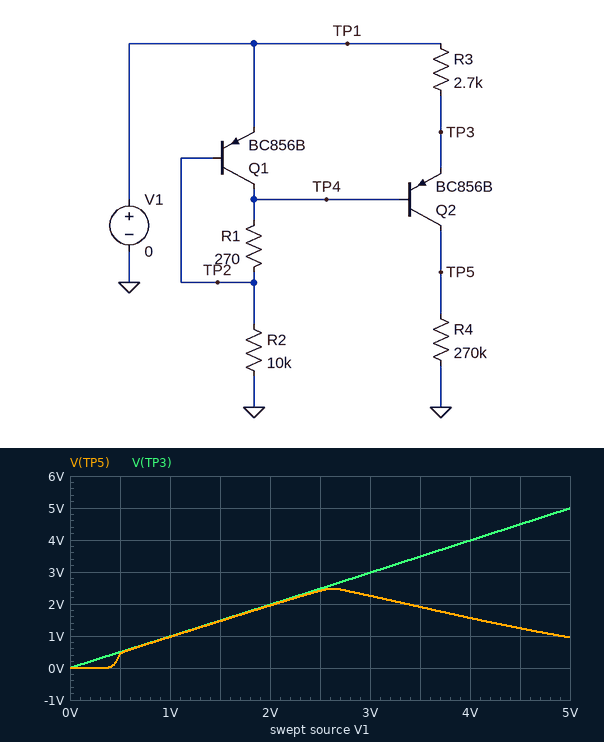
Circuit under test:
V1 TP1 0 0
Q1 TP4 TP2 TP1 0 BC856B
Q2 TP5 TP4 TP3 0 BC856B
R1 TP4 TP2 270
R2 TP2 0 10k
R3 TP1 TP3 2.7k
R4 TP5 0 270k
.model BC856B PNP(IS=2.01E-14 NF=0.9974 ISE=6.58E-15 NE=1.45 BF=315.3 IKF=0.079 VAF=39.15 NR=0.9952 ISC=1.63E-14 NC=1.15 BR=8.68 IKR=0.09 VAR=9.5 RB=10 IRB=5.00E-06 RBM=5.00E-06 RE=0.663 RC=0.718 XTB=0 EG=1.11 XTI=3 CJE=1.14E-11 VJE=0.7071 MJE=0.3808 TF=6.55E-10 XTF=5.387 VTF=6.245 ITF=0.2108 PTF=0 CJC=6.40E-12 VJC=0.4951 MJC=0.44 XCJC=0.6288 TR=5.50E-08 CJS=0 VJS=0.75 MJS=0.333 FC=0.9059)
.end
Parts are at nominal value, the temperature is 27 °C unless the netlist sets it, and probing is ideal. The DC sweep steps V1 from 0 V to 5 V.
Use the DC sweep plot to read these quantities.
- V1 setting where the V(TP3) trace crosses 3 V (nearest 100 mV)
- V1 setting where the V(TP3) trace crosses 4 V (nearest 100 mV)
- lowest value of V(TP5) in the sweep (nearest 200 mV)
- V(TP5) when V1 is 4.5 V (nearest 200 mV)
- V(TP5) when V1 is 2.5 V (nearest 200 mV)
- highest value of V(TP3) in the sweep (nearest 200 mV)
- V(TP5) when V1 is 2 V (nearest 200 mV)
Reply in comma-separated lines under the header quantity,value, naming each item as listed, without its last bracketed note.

quantity,value
V1 setting where the V(TP3) trace crosses 3 V,3.0 V
V1 setting where the V(TP3) trace crosses 4 V,4.0 V
lowest value of V(TP5) in the sweep,0 V
V(TP5) when V1 is 4.5 V,1.2 V
V(TP5) when V1 is 2.5 V,2.4 V
highest value of V(TP3) in the sweep,5.0 V
V(TP5) when V1 is 2 V,2.0 V
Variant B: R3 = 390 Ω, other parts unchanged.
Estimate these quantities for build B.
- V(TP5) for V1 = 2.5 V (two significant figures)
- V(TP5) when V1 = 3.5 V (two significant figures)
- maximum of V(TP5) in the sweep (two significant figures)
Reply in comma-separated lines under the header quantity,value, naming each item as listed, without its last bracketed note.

quantity,value
V(TP5) for V1 = 2.5 V,2.5 V
V(TP5) when V1 = 3.5 V,3.2 V
maximum of V(TP5) in the sweep,3.3 V
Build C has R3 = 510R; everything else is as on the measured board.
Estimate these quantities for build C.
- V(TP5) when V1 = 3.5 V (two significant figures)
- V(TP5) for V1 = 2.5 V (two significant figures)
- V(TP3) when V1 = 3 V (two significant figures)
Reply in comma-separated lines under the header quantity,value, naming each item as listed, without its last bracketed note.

quantity,value
V(TP5) when V1 = 3.5 V,3.1 V
V(TP5) for V1 = 2.5 V,2.5 V
V(TP3) when V1 = 3 V,3.0 V
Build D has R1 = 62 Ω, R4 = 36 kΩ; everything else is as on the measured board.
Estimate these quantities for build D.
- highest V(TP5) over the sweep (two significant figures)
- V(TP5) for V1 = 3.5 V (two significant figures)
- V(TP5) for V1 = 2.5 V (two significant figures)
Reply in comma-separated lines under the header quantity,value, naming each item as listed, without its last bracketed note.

quantity,value
highest V(TP5) over the sweep,730 mV
V(TP5) for V1 = 3.5 V,710 mV
V(TP5) for V1 = 2.5 V,660 mV
